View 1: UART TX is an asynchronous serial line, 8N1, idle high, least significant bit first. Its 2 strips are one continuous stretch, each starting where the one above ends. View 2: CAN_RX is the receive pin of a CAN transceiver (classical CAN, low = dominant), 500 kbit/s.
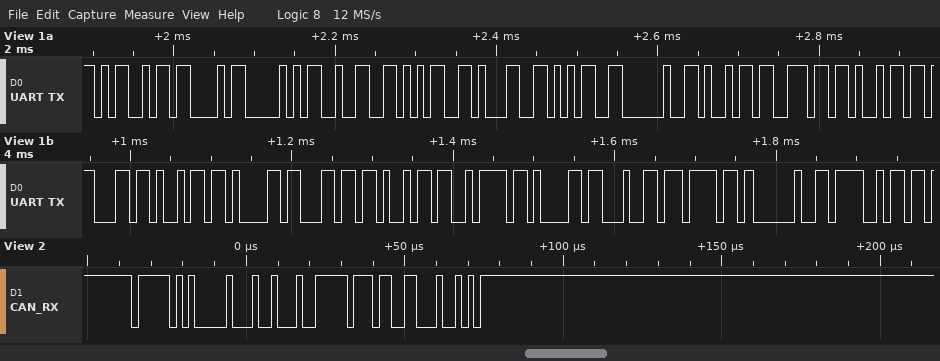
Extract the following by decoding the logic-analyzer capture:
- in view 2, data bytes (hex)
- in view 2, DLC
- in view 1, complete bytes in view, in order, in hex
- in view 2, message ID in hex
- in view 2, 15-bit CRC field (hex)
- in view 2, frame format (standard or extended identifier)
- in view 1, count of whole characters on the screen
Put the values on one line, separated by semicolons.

44 FF; 2; 4D 43 50 32 35 31 35 20 69 6E 69 63 69 61 6C 69 7A 61 64 6F 20 4F; 0x7E8; 0x3312; standard; 22
